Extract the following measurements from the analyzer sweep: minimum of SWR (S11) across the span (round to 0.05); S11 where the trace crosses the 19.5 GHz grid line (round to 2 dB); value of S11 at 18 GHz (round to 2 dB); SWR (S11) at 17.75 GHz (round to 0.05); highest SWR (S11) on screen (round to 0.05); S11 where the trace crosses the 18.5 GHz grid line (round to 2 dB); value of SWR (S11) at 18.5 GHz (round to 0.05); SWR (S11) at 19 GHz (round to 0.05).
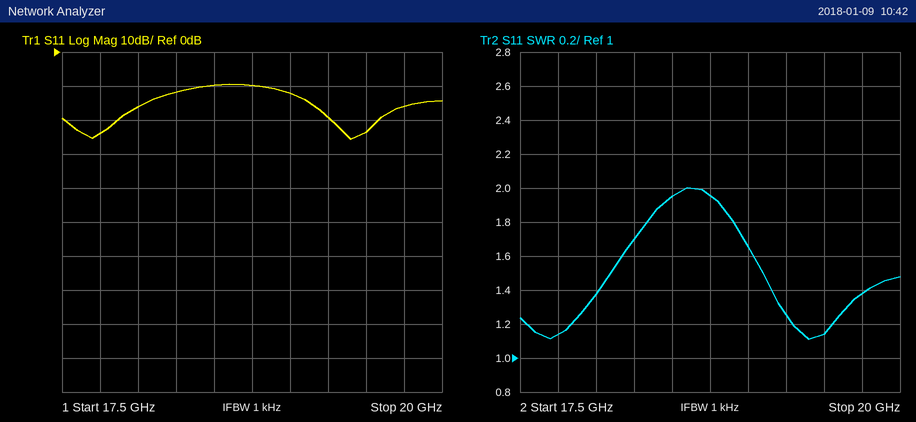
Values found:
1.10
-24 dB
-16 dB
1.15
2.00
-10 dB
1.95
1.65
